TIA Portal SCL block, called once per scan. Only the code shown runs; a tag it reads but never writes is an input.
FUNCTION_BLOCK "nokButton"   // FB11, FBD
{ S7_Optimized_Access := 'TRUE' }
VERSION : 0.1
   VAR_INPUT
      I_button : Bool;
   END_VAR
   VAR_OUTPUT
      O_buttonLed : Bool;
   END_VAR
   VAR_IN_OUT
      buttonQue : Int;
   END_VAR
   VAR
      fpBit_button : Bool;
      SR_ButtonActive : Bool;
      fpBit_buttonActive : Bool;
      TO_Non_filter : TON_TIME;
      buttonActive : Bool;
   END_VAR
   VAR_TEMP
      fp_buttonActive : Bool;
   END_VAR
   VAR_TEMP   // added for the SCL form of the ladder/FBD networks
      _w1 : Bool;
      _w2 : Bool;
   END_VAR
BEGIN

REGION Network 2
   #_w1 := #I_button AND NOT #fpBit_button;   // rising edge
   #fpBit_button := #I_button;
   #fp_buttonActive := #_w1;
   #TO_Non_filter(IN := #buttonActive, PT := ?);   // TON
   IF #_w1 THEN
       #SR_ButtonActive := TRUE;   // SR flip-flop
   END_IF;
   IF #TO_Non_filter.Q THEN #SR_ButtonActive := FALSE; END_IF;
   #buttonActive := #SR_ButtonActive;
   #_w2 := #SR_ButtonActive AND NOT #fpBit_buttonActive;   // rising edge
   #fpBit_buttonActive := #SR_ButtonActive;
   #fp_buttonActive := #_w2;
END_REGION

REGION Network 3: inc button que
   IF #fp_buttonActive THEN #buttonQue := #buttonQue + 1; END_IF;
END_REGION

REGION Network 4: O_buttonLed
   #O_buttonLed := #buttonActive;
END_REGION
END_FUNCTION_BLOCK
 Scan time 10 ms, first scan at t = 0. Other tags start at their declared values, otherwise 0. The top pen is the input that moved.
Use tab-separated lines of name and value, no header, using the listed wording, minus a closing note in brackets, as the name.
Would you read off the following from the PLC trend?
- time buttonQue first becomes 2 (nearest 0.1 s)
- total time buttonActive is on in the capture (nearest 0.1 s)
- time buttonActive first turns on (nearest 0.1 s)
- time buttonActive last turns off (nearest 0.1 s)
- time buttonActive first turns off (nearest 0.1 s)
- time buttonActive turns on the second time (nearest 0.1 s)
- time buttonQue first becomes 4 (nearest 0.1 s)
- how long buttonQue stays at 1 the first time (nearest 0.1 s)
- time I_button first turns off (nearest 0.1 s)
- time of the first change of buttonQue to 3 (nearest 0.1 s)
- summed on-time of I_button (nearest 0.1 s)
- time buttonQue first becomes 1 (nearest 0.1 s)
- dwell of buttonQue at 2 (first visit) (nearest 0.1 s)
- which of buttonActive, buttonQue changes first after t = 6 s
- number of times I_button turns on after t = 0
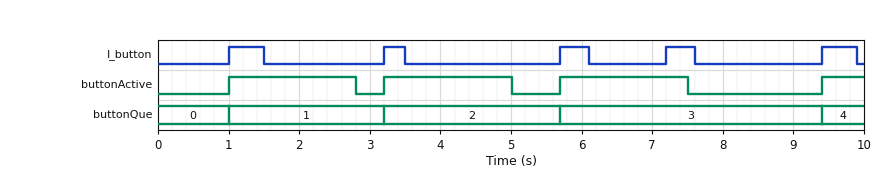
time buttonQue first becomes 2	3.2 s
total time buttonActive is on in the capture	6.0 s
time buttonActive first turns on	1.0 s
time buttonActive last turns off	7.5 s
time buttonActive first turns off	2.8 s
time buttonActive turns on the second time	3.2 s
time buttonQue first becomes 4	9.4 s
how long buttonQue stays at 1 the first time	2.2 s
time I_button first turns off	1.5 s
time of the first change of buttonQue to 3	5.7 s
summed on-time of I_button	2.1 s
time buttonQue first becomes 1	1.0 s
dwell of buttonQue at 2 (first visit)	2.5 s
which of buttonActive, buttonQue changes first after t = 6 s	buttonActive
number of times I_button turns on after t = 0	5
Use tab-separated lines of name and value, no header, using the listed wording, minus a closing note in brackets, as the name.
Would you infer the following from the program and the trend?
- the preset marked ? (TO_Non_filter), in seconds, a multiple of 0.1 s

the preset marked ? (TO_Non_filter), in seconds, a multiple of 0.1 s	1.8 s
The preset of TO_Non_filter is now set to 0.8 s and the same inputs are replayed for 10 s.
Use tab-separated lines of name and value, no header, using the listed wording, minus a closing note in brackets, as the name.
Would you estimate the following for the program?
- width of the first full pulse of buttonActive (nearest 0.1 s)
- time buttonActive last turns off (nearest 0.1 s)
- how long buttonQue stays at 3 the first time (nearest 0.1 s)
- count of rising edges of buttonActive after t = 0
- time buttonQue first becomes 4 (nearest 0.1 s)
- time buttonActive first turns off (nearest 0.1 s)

width of the first full pulse of buttonActive	0.8 s
time buttonActive last turns off	8.0 s
how long buttonQue stays at 3 the first time	1.5 s
count of rising edges of buttonActive after t = 0	5
time buttonQue first becomes 4	7.2 s
time buttonActive first turns off	1.8 s
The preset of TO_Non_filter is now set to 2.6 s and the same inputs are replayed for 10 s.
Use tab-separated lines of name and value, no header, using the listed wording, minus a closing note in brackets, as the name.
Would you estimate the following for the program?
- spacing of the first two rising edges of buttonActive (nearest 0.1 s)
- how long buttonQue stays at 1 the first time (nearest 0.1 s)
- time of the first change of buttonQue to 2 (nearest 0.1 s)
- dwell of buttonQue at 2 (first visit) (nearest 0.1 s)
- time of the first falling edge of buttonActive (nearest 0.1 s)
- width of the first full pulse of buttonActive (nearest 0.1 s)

spacing of the first two rising edges of buttonActive	4.7 s
how long buttonQue stays at 1 the first time	4.7 s
time of the first change of buttonQue to 2	5.7 s
dwell of buttonQue at 2 (first visit)	3.7 s
time of the first falling edge of buttonActive	3.6 s
width of the first full pulse of buttonActive	2.6 s
